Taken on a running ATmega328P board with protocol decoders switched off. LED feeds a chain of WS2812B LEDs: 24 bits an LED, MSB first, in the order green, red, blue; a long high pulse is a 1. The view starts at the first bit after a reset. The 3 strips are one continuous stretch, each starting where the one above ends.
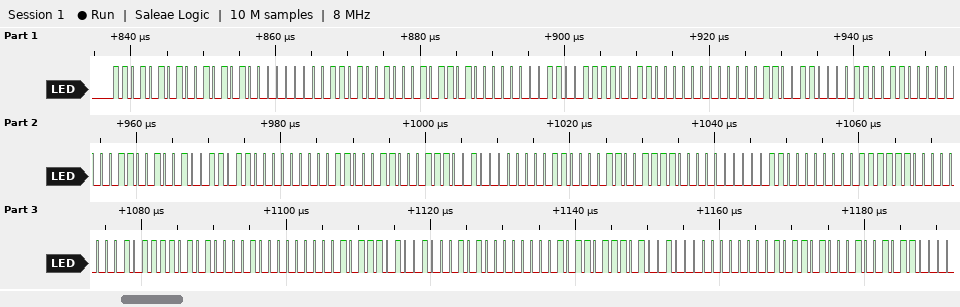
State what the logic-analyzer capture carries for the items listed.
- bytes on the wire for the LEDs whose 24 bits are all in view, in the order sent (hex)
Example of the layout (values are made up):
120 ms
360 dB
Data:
D5 2A 00 D2 2D 00 CF 30 00 CC 33 00 C9 36 00 C6 39 00 C3 3C 00 C0 3F 00 BD 42 00 BA 45 00 B7 48 00
